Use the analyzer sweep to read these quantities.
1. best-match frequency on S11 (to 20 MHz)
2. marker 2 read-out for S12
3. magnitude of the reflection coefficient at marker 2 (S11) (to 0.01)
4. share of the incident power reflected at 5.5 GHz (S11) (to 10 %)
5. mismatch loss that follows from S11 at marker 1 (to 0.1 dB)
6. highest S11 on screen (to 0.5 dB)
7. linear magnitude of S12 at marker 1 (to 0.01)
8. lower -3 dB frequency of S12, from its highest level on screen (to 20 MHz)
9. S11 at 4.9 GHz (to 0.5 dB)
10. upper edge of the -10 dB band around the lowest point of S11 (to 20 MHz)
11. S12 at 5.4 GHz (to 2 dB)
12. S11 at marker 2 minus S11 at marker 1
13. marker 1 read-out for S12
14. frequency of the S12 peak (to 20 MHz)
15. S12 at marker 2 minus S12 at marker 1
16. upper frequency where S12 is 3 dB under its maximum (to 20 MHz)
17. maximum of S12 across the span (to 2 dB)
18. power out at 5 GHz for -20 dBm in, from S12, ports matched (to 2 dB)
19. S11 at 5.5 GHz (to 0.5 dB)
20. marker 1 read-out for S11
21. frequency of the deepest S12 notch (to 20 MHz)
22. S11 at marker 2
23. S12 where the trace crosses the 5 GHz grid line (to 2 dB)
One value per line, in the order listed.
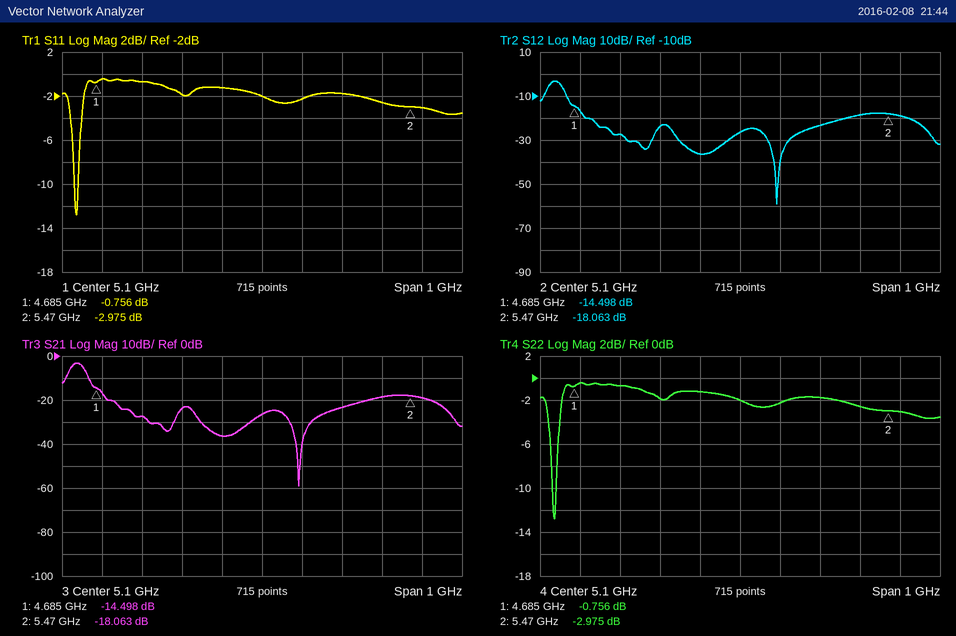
4.64 GHz
-18.063 dB
0.71
50 %
8.0 dB
-0.5 dB
0.19
4.62 GHz
-2.0 dB
4.64 GHz
-18 dB
-2.219 dB
-14.498 dB
4.64 GHz
-3.565 dB
4.66 GHz
-4 dB
-56 dBm
-3.0 dB
-0.756 dB
5.20 GHz
-2.975 dB
-36 dB
